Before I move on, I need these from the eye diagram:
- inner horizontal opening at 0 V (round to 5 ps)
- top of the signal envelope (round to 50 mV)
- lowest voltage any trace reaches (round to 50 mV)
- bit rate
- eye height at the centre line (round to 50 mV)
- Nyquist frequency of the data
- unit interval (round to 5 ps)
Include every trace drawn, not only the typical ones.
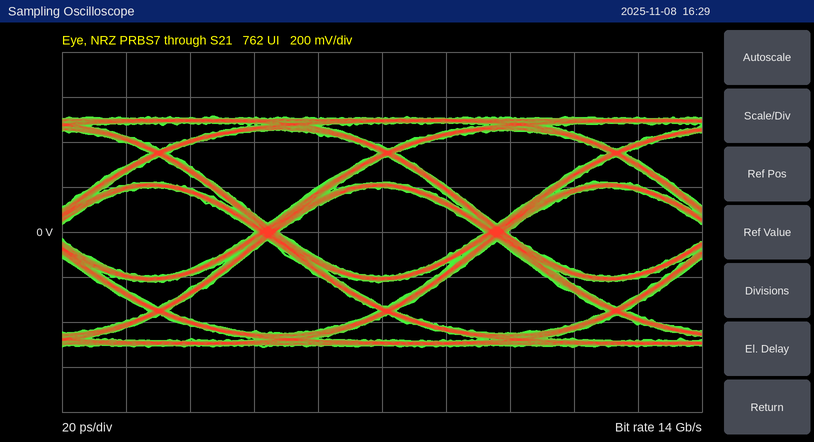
65 ps
500 mV
-500 mV
14 Gb/s
400 mV
7 GHz
70 ps
